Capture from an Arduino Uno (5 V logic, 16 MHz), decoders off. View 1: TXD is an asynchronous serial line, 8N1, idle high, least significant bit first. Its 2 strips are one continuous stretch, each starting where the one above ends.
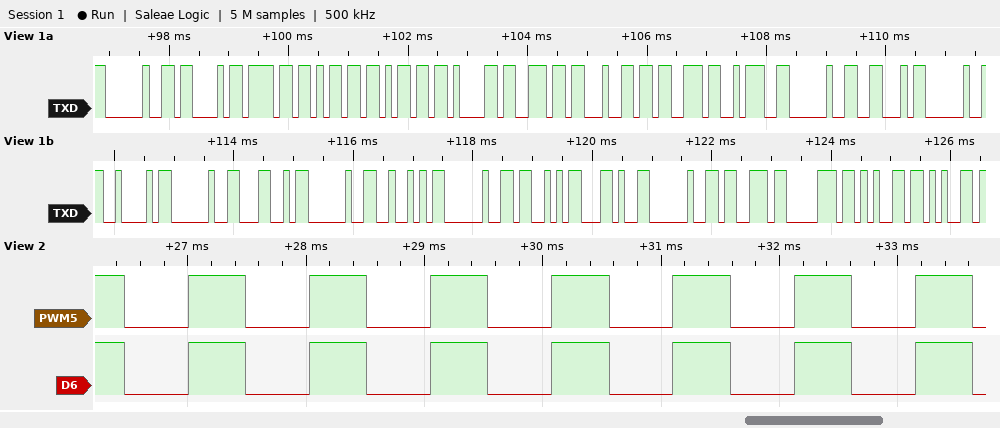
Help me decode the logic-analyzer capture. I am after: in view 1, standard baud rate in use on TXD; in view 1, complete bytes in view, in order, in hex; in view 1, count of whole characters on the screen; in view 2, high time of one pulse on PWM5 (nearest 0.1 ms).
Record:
9600 baud
20 43 6F 6D 6D 61 6E 64 73 3A 20 46 20 42 20 4C 20 52 20 53 2C 20 73 70 65 65
26
0.5 ms
